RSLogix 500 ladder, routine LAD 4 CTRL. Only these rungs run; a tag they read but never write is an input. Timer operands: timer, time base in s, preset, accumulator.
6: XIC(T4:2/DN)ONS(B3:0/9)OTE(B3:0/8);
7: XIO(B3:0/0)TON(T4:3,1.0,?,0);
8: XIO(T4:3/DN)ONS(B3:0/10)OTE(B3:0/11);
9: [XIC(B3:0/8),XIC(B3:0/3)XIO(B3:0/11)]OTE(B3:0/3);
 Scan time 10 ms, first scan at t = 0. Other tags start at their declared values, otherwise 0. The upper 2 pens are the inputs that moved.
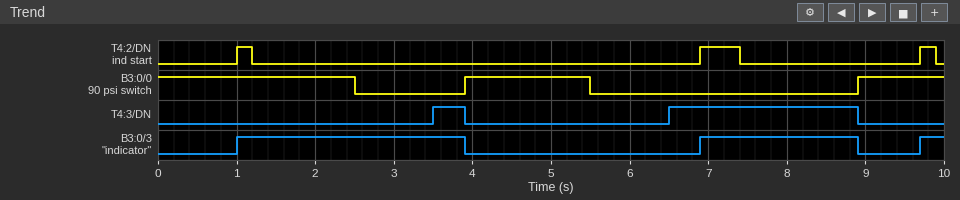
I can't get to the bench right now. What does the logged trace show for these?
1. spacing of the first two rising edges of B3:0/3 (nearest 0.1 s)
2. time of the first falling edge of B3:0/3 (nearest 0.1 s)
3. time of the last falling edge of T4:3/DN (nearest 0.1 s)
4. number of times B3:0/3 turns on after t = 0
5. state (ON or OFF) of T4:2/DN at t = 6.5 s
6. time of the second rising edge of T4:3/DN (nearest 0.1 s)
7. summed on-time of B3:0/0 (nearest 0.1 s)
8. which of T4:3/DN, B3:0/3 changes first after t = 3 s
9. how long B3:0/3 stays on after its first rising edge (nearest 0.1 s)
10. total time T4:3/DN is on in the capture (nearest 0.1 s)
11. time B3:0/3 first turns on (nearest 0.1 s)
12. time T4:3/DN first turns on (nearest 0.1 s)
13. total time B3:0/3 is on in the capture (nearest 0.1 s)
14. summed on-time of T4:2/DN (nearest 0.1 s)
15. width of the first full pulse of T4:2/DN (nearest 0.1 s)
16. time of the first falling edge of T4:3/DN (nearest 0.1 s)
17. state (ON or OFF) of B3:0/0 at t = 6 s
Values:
5.9 s
3.9 s
8.9 s
3
OFF
6.5 s
5.2 s
T4:3/DN
2.9 s
2.8 s
1.0 s
3.5 s
5.2 s
0.9 s
0.2 s
3.9 s
OFF
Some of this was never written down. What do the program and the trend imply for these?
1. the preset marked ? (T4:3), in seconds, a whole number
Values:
1 s
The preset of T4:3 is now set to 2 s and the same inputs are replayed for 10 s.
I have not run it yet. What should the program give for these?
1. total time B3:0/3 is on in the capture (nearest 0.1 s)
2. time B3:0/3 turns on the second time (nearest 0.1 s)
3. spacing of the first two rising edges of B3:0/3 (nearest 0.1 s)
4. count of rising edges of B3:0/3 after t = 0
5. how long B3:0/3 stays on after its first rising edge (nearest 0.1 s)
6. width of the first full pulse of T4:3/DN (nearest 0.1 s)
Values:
8.2 s
9.7 s
8.7 s
2
7.9 s
1.4 s
